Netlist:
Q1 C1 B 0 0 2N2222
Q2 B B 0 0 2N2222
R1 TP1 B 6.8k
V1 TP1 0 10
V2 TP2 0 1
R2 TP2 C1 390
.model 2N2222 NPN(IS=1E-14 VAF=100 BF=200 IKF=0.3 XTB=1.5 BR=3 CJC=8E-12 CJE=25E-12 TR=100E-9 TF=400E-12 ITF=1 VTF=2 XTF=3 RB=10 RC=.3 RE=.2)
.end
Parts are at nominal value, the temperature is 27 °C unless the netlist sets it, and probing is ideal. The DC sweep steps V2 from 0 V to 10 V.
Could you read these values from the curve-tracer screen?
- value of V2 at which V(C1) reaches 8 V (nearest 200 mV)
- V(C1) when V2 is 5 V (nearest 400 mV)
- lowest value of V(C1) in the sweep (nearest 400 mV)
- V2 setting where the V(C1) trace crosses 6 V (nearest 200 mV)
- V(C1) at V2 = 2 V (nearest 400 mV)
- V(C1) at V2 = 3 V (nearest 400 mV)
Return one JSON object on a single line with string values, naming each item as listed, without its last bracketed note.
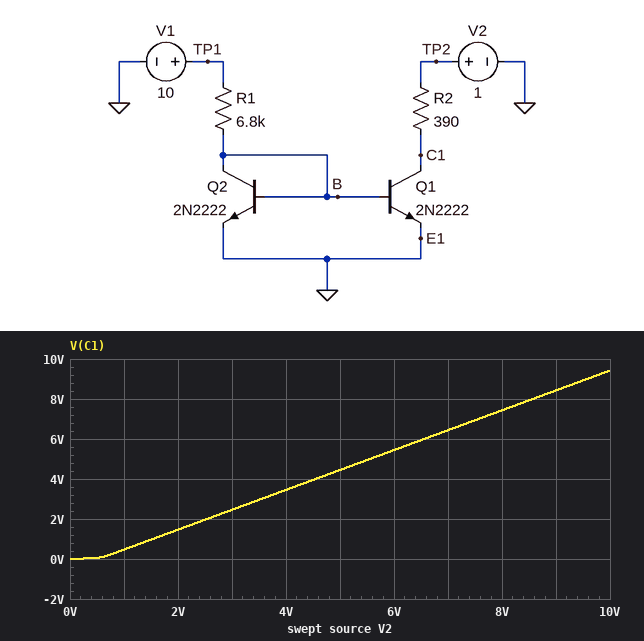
{"value of V2 at which V(C1) reaches 8 V": "8.6 V", "V(C1) when V2 is 5 V": "4.4 V", "lowest value of V(C1) in the sweep": "0 V", "V2 setting where the V(C1) trace crosses 6 V": "6.6 V", "V(C1) at V2 = 2 V": "1.6 V", "V(C1) at V2 = 3 V": "2.4 V"}
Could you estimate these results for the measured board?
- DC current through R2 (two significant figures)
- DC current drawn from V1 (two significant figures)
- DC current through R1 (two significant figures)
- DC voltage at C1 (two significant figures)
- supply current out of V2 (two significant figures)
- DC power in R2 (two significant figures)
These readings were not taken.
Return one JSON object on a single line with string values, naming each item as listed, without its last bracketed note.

{"DC current through R2": "1.4 mA", "DC current drawn from V1": "1.4 mA", "DC current through R1": "1.4 mA", "DC voltage at C1": "470 mV", "supply current out of V2": "1.4 mA", "DC power in R2": "720 µW"}
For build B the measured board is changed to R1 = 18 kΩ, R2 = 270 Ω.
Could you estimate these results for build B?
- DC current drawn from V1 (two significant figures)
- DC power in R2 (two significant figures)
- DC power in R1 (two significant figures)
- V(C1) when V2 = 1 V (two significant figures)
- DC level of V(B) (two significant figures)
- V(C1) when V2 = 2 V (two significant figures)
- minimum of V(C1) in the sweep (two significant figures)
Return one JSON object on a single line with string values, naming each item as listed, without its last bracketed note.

{"DC current drawn from V1": "520 µA", "DC power in R2": "72 µW", "DC power in R1": "4.9 mW", "V(C1) when V2 = 1 V": "860 mV", "DC level of V(B)": "640 mV", "V(C1) when V2 = 2 V": "1.9 V", "minimum of V(C1) in the sweep": "6.1 mV"}
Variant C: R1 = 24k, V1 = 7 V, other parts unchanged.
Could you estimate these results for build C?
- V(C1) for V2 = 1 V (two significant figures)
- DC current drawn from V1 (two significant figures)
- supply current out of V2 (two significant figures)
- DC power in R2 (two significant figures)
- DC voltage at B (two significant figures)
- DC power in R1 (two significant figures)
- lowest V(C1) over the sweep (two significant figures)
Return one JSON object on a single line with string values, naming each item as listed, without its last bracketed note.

{"V(C1) for V2 = 1 V": "900 mV", "DC current drawn from V1": "270 µA", "supply current out of V2": "260 µA", "DC power in R2": "27 µW", "DC voltage at B": "620 mV", "DC power in R1": "1.7 mW", "lowest V(C1) over the sweep": "5.7 mV"}
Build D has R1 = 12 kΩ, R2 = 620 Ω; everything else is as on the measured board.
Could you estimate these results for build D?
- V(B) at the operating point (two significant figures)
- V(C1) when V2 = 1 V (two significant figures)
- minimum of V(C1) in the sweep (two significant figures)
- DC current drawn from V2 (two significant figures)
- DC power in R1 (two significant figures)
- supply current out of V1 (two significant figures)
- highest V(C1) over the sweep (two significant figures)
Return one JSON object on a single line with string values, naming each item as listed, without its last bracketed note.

{"V(B) at the operating point": "650 mV", "V(C1) when V2 = 1 V": "520 mV", "minimum of V(C1) in the sweep": "7.0 mV", "DC current drawn from V2": "770 µA", "DC power in R1": "7.3 mW", "supply current out of V1": "780 µA", "highest V(C1) over the sweep": "9.5 V"}
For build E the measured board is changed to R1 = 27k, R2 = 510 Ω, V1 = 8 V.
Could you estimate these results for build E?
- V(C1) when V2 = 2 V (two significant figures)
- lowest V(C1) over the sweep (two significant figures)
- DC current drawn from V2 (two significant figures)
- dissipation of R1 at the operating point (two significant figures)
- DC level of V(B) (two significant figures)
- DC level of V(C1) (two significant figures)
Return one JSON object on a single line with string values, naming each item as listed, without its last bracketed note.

{"V(C1) when V2 = 2 V": "1.9 V", "lowest V(C1) over the sweep": "6.1 mV", "DC current drawn from V2": "270 µA", "dissipation of R1 at the operating point": "2.0 mW", "DC level of V(B)": "620 mV", "DC level of V(C1)": "860 mV"}
